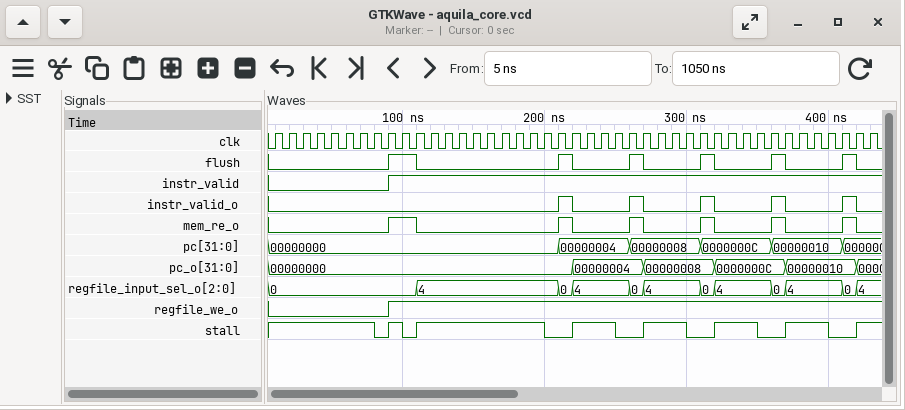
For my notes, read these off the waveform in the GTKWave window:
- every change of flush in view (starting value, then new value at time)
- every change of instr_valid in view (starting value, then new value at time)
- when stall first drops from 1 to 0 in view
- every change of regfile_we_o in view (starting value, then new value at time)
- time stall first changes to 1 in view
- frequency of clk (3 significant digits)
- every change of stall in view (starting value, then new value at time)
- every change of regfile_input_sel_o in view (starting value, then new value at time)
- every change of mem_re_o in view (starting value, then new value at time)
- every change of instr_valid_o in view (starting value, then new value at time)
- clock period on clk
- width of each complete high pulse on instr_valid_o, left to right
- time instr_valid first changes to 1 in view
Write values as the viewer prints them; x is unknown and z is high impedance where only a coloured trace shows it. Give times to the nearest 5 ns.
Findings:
0, 1 at 90 ns, 0 at 110 ns, 1 at 210 ns, 0 at 220 ns, 1 at 260 ns, 0 at 270 ns, 1 at 310 ns, 0 at 320 ns, 1 at 360 ns, 0 at 370 ns, 1 at 410 ns, 0 at 420 ns
0, 1 at 90 ns
80 ns
0, 1 at 90 ns
90 ns
100 MHz
1, 0 at 80 ns, 1 at 90 ns, 0 at 100 ns, 1 at 110 ns, 0 at 200 ns, 1 at 220 ns, 0 at 250 ns, 1 at 270 ns, 0 at 300 ns, 1 at 320 ns, 0 at 350 ns, 1 at 370 ns, 0 at 400 ns, 1 at 420 ns
0, 4 at 110 ns, 0 at 210 ns, 4 at 220 ns, 0 at 260 ns, 4 at 270 ns, 0 at 310 ns, 4 at 320 ns, 0 at 360 ns, 4 at 370 ns, 0 at 410 ns, 4 at 420 ns
0, 1 at 90 ns, 0 at 110 ns, 1 at 210 ns, 0 at 220 ns, 1 at 260 ns, 0 at 270 ns, 1 at 310 ns, 0 at 320 ns, 1 at 360 ns, 0 at 370 ns, 1 at 410 ns, 0 at 420 ns
0, 1 at 210 ns, 0 at 220 ns, 1 at 260 ns, 0 at 270 ns, 1 at 310 ns, 0 at 320 ns, 1 at 360 ns, 0 at 370 ns, 1 at 410 ns, 0 at 420 ns
10 ns
10 ns, 10 ns, 10 ns, 10 ns, 10 ns
90 ns
